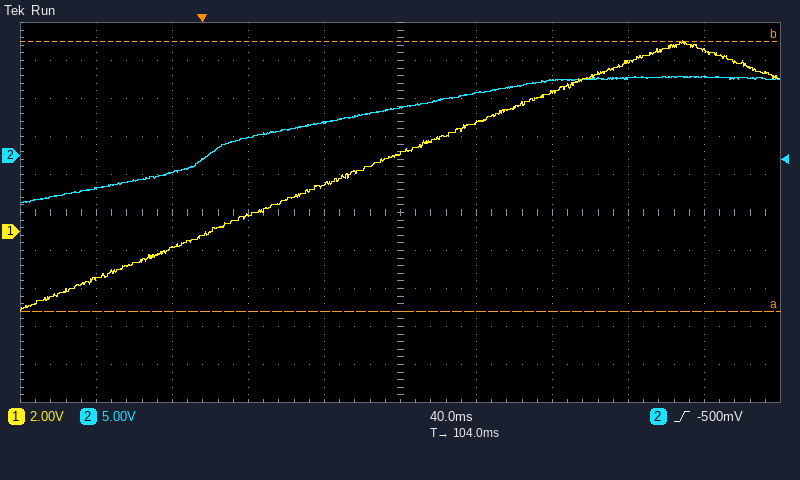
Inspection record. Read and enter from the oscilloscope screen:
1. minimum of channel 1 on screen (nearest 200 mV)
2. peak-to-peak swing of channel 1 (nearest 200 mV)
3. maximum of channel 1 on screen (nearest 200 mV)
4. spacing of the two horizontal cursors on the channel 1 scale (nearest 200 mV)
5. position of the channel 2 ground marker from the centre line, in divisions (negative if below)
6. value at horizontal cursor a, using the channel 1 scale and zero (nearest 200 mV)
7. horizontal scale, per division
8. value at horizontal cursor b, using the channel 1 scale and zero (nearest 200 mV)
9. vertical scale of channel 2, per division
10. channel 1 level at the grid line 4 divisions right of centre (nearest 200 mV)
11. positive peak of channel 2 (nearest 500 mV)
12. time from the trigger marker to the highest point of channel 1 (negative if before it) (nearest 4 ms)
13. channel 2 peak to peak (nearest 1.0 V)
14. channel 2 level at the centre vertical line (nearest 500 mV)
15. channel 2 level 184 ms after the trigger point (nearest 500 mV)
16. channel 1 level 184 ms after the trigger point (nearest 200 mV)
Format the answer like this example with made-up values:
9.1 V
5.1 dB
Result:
-4.2 V
14.2 V
10.0 V
14.2 V
+1.5 div
-4.2 V
40 ms
10.0 V
5 V
9.6 V
10.5 V
+252 ms
17.0 V
6.5 V
10.0 V
7.4 V
